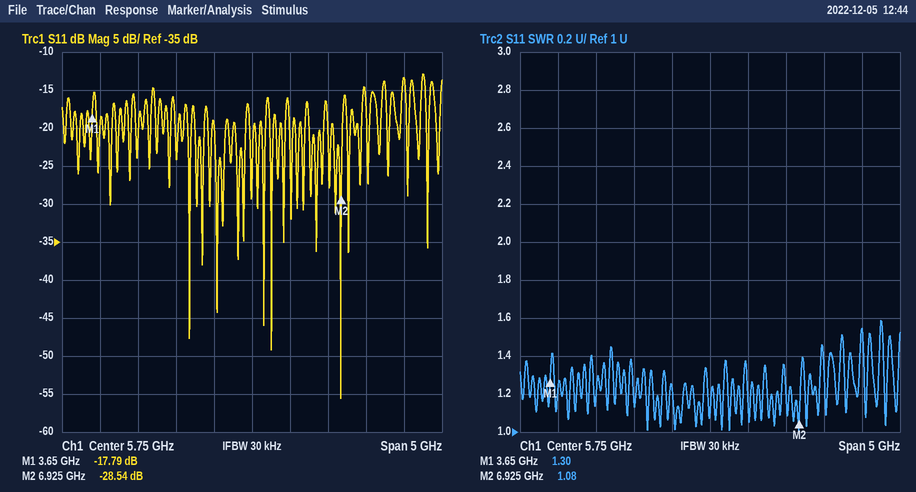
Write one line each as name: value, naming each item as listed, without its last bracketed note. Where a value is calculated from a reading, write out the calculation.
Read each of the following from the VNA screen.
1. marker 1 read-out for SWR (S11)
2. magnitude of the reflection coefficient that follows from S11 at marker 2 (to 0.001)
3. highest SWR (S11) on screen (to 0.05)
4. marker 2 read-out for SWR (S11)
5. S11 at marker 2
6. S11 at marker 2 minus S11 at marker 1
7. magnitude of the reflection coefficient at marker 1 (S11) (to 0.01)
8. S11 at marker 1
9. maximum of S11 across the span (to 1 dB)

marker 1 read-out for SWR: 1.30
magnitude of the reflection coefficient that follows from S11 at marker 2: 10^(-28.54/20) ≈ 0.037
highest SWR (S11) on screen: 1.60
marker 2 read-out for SWR: 1.08
S11 at marker 2: -28.54 dB
S11 at marker 2 minus S11 at marker 1: -28.54 − (-17.79) = -10.75 dB
magnitude of the reflection coefficient at marker 1 (S11): 10^(-17.79/20) ≈ 0.13
S11 at marker 1: -17.79 dB
maximum of S11 across the span: -13 dB
